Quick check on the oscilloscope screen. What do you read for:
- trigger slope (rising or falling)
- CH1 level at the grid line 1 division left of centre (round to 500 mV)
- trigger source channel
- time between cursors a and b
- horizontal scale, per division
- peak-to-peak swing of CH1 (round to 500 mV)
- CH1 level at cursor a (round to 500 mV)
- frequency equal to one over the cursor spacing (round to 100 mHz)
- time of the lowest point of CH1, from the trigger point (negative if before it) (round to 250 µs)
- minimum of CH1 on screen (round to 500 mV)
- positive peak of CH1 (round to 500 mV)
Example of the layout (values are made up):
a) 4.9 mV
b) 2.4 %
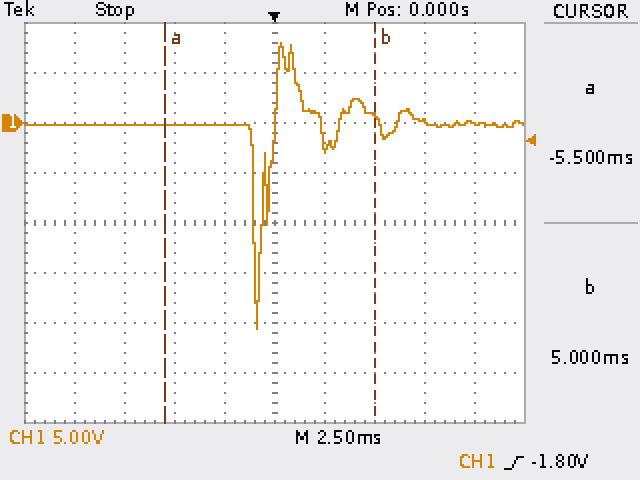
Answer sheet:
a) rising
b) 0.0 V
c) CH1
d) 10.50 ms
e) 2.5 ms
f) 28.5 V
g) 0.0 V
h) 95.2 Hz
i) -750 µs
j) -20.5 V
k) 8.0 V
